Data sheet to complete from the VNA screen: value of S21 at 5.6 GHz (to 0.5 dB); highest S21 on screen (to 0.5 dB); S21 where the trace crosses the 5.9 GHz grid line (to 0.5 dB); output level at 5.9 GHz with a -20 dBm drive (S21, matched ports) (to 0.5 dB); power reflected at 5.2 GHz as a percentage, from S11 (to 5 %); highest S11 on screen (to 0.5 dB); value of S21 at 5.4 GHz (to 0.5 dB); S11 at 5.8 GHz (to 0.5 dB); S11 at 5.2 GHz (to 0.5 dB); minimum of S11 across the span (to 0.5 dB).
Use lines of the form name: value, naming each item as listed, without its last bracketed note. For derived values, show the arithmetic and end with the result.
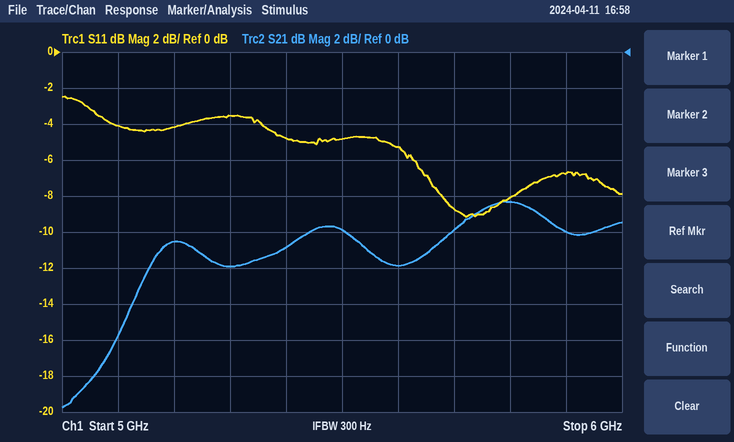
value of S21 at 5.6 GHz: -12.0 dB
highest S21 on screen: -8.5 dB
S21 where the trace crosses the 5.9 GHz grid line: -10.0 dB
output level at 5.9 GHz with a -20 dBm drive (S21, matched ports): -20 dBm + (-10.0 dB) = -30.0 dBm
power reflected at 5.2 GHz as a percentage, from S11: 10^(-4/10) ≈ 40 %
highest S11 on screen: -2.5 dB
value of S21 at 5.4 GHz: -11.0 dB
S11 at 5.8 GHz: -8.0 dB
S11 at 5.2 GHz: -4.0 dB
minimum of S11 across the span: -9.0 dB
